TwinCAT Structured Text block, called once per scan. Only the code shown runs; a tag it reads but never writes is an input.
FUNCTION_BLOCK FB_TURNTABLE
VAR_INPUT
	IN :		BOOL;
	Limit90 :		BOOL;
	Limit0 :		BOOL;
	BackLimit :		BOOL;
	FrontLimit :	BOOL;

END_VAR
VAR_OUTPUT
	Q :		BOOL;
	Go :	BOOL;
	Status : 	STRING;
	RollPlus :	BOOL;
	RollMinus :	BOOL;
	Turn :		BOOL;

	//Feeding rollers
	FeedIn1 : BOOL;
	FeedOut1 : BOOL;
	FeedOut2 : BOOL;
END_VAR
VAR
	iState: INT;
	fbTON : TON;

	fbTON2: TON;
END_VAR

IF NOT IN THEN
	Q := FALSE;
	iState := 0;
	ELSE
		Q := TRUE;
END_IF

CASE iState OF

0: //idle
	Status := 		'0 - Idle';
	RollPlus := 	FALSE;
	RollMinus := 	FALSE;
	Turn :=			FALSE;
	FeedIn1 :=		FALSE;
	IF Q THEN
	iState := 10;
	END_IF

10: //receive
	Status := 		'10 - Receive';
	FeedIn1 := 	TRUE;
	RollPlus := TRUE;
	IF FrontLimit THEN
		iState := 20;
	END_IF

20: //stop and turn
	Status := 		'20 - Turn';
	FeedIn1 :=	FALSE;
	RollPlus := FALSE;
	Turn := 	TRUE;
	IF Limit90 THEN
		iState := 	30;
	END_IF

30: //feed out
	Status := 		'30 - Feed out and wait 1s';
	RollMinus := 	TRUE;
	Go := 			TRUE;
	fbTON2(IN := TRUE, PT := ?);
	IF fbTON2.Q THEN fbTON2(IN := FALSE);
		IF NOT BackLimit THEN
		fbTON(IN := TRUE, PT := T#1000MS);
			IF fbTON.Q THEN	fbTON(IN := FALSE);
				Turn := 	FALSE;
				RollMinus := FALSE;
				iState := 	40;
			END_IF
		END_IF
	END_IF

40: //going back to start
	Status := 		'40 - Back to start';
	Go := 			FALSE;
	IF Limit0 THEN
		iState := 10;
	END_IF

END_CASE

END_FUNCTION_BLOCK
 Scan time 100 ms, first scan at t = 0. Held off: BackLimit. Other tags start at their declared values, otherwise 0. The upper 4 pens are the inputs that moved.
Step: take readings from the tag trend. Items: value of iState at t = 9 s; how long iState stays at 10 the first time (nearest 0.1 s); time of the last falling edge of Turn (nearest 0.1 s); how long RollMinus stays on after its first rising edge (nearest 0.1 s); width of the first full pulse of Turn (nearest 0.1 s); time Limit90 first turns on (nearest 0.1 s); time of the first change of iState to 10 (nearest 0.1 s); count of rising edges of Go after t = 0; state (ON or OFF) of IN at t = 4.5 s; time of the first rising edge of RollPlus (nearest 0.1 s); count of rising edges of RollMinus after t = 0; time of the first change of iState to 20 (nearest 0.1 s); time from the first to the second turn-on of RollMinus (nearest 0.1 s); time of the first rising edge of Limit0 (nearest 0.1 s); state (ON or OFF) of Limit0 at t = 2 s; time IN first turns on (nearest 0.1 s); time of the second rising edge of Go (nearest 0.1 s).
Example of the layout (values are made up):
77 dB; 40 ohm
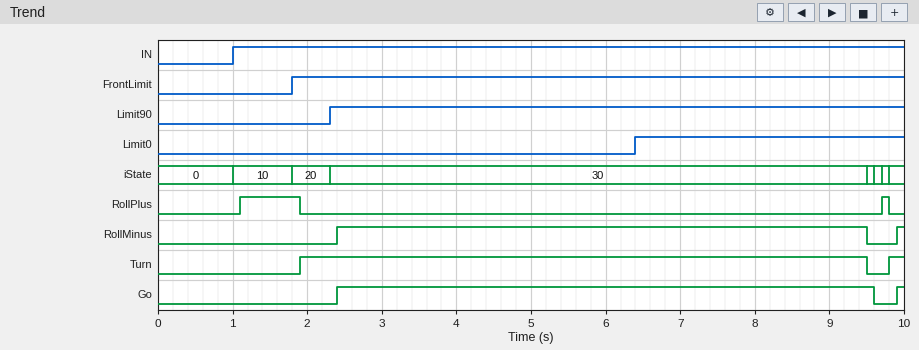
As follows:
30; 0.8 s; 9.5 s; 7.1 s; 7.6 s; 2.3 s; 1.0 s; 2; ON; 1.1 s; 2; 1.8 s; 7.5 s; 6.4 s; OFF; 1.0 s; 9.9 s
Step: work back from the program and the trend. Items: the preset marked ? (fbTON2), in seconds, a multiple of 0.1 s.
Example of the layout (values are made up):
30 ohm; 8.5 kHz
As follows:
3.5 s
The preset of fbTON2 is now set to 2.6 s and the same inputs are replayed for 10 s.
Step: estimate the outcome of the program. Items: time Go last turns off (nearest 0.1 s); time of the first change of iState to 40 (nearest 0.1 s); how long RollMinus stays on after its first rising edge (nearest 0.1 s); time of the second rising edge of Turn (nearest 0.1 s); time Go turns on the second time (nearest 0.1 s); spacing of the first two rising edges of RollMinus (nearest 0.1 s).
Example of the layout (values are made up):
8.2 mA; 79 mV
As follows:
7.8 s; 7.7 s; 5.3 s; 8.0 s; 8.1 s; 5.7 s
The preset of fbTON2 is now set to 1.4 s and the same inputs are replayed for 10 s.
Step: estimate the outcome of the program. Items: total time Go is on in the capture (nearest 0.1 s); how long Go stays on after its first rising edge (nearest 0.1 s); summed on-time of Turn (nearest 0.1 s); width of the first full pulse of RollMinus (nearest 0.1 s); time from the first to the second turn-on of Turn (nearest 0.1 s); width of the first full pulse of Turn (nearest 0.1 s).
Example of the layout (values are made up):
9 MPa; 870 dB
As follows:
6.0 s; 3.0 s; 6.5 s; 2.9 s; 4.7 s; 3.4 s
